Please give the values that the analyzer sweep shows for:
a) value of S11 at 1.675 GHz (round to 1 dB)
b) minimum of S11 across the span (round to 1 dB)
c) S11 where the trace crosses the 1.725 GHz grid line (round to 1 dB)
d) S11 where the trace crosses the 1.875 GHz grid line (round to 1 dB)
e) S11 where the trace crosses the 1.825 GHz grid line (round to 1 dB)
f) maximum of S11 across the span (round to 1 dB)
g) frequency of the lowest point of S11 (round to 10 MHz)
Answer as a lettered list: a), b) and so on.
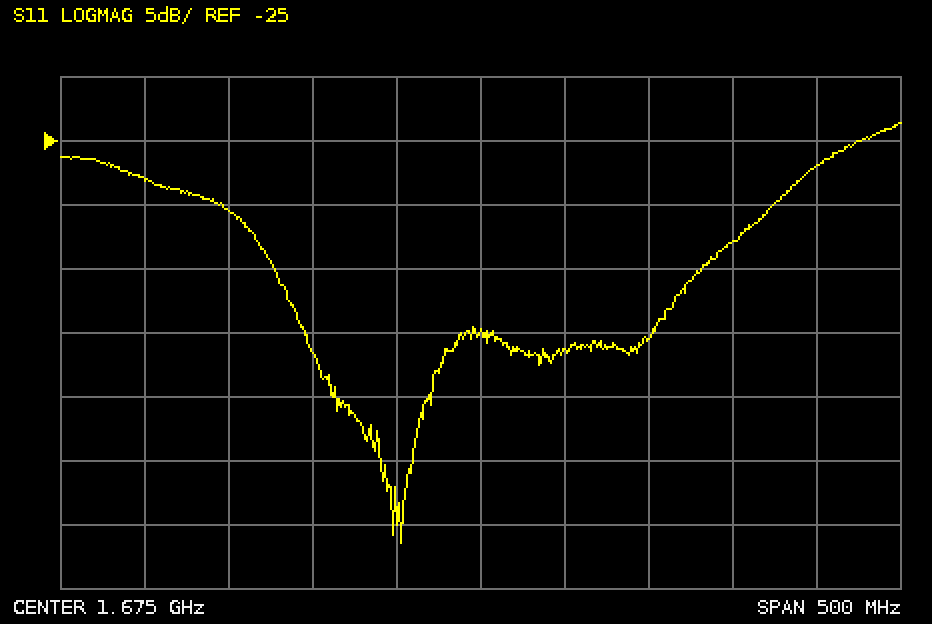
a) -40 dB
b) -56 dB
c) -41 dB
d) -27 dB
e) -33 dB
f) -24 dB
g) 1.63 GHz
